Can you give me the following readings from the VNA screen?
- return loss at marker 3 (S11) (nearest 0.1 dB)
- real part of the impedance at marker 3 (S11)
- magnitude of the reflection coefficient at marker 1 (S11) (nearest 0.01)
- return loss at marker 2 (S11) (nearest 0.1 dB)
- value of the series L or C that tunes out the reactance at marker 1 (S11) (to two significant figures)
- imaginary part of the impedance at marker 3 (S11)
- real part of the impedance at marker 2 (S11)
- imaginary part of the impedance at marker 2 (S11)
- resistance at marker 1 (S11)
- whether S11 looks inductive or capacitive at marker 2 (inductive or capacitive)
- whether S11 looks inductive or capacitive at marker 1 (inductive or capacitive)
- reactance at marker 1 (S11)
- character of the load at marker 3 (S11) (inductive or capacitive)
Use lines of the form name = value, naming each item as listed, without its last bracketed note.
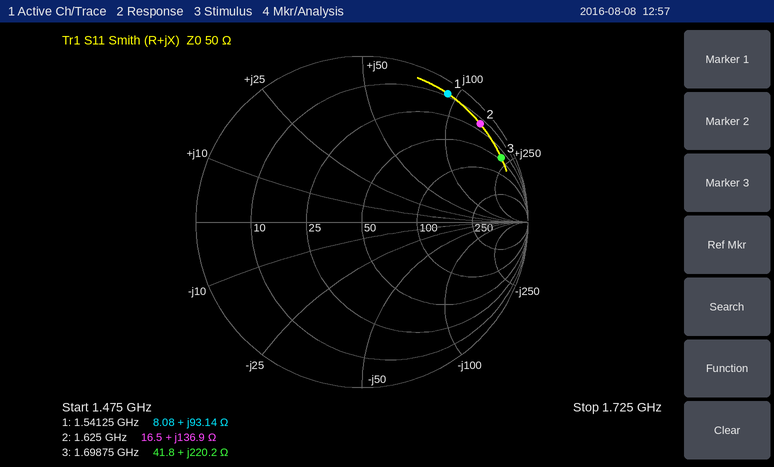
return loss at marker 3 (S11) = 0.7 dB
real part of the impedance at marker 3 = 41.8 Ω
magnitude of the reflection coefficient at marker 1 (S11) = 0.93
return loss at marker 2 (S11) = 0.7 dB
value of the series L or C that tunes out the reactance at marker 1 (S11) = 1.1 pF
imaginary part of the impedance at marker 3 = +220.2 Ω
real part of the impedance at marker 2 = 16.5 Ω
imaginary part of the impedance at marker 2 = +136.9 Ω
resistance at marker 1 = 8.08 Ω
whether S11 looks inductive or capacitive at marker 2 = inductive
whether S11 looks inductive or capacitive at marker 1 = inductive
reactance at marker 1 = +93.14 Ω
character of the load at marker 3 (S11) = inductive
